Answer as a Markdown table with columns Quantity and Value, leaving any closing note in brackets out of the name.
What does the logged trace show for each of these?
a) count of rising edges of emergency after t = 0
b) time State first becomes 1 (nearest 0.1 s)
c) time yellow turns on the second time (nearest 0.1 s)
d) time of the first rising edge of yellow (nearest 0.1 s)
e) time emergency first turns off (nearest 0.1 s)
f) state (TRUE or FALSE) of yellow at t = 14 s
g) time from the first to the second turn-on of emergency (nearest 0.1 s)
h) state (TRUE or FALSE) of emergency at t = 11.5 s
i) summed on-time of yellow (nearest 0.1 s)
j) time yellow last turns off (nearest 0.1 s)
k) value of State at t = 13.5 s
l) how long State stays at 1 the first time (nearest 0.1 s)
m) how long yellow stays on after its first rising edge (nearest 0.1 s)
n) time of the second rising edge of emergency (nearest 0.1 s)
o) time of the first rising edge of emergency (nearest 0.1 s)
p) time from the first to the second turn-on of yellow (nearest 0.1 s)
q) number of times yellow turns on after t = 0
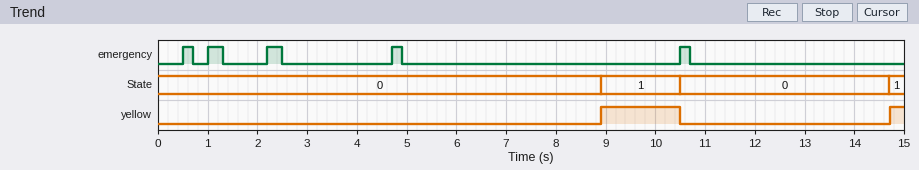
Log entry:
| Quantity | Value |
|---|---|
| count of rising edges of emergency after t = 0 | 5 |
| time State first becomes 1 | 8.9 s |
| time yellow turns on the second time | 14.7 s |
| time of the first rising edge of yellow | 8.9 s |
| time emergency first turns off | 0.7 s |
| state (TRUE or FALSE) of yellow at t = 14 s | FALSE |
| time from the first to the second turn-on of emergency | 0.5 s |
| state (TRUE or FALSE) of emergency at t = 11.5 s | FALSE |
| summed on-time of yellow | 1.9 s |
| time yellow last turns off | 10.5 s |
| value of State at t = 13.5 s | 0 |
| how long State stays at 1 the first time | 1.6 s |
| how long yellow stays on after its first rising edge | 1.6 s |
| time of the second rising edge of emergency | 1.0 s |
| time of the first rising edge of emergency | 0.5 s |
| time from the first to the second turn-on of yellow | 5.8 s |
| number of times yellow turns on after t = 0 | 2 |
